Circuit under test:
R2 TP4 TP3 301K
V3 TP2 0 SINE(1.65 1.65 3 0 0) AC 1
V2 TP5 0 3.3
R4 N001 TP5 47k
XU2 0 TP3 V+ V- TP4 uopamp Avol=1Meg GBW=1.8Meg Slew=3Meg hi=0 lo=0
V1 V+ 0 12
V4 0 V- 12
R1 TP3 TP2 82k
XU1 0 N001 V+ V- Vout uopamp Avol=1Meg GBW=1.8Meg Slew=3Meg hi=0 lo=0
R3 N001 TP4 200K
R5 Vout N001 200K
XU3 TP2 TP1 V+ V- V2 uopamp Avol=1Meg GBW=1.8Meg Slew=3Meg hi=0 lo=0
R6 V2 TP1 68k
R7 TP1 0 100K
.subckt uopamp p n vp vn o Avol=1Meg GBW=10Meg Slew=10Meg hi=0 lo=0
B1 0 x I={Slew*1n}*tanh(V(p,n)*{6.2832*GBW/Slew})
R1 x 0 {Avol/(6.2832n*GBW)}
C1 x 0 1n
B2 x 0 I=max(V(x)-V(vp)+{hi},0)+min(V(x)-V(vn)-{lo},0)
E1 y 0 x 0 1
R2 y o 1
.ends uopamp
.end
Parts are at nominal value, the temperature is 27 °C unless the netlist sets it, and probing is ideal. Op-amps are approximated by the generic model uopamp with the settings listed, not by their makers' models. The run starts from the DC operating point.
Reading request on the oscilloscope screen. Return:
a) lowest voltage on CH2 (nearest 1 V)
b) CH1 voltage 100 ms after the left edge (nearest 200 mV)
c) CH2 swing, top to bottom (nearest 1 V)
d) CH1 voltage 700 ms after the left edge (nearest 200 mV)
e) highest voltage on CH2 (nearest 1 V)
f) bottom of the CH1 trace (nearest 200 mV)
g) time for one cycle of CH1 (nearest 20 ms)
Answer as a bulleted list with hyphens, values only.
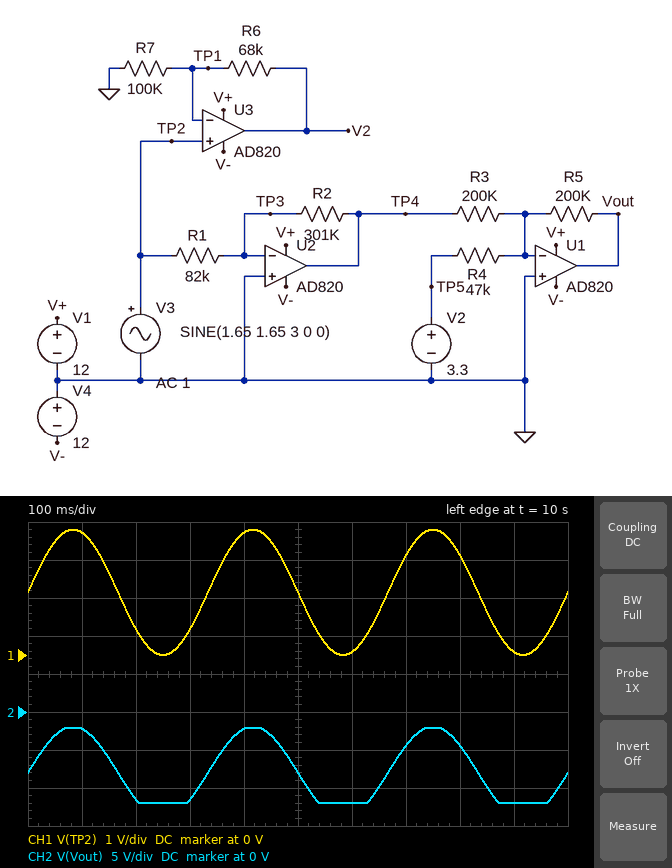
- -12 V
- 3.2 V
- 10 V
- 2.6 V
- -2 V
- 0 V
- 340 ms
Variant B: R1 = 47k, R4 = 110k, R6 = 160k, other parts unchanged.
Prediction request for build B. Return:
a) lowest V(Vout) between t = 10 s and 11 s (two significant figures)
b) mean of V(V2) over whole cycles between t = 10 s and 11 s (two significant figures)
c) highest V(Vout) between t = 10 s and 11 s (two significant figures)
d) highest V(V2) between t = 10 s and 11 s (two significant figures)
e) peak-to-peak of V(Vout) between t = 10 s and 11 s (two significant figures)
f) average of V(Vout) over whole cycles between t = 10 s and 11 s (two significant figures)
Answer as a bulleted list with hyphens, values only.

- -6.0 V
- 4.3 V
- 6.0 V
- 8.6 V
- 12 V
- 1.9 V
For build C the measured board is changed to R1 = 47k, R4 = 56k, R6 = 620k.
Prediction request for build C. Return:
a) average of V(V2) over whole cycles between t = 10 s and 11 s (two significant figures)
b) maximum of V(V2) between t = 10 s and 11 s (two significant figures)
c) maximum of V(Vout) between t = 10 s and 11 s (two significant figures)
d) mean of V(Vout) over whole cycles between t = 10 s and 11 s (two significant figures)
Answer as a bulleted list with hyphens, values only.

- 8.2 V
- 12 V
- 220 mV
- -3.9 V
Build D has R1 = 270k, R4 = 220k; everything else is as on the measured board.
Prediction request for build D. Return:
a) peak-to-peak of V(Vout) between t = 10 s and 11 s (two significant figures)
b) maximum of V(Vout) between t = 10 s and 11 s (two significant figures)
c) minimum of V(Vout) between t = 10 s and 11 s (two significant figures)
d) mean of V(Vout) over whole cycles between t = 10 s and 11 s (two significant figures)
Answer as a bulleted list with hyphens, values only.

- 3.7 V
- 680 mV
- -3.0 V
- -1.2 V
